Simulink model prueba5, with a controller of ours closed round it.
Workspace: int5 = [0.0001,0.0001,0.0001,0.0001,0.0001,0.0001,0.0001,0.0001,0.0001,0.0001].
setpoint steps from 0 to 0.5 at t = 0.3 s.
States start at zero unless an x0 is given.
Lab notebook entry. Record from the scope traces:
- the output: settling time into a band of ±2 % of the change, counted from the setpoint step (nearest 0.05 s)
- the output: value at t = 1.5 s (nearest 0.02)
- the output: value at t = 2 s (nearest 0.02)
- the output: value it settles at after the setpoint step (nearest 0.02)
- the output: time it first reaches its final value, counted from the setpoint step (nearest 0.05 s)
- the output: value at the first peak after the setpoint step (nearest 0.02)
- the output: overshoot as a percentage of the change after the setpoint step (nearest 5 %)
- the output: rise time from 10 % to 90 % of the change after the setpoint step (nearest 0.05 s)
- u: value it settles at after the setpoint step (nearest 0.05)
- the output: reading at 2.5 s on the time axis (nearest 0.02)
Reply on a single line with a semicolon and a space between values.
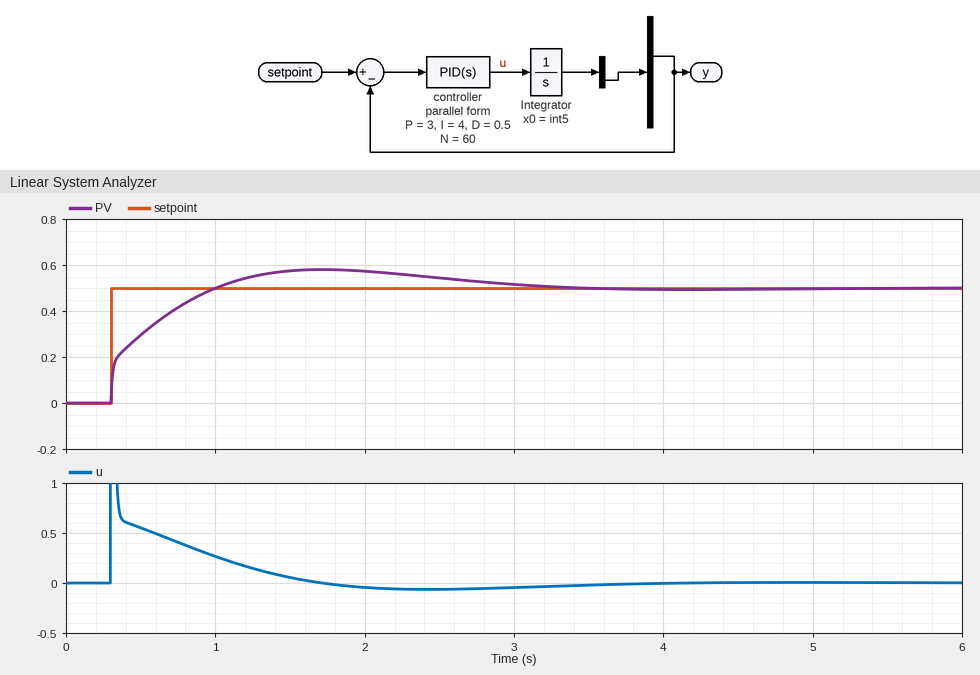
2.85 s; 0.58; 0.58; 0.50; 0.70 s; 0.58; 15 %; 0.55 s; 0.00; 0.54
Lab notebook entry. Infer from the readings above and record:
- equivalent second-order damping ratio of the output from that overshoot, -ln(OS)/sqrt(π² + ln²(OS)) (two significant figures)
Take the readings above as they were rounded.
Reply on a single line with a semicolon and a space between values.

0.52
